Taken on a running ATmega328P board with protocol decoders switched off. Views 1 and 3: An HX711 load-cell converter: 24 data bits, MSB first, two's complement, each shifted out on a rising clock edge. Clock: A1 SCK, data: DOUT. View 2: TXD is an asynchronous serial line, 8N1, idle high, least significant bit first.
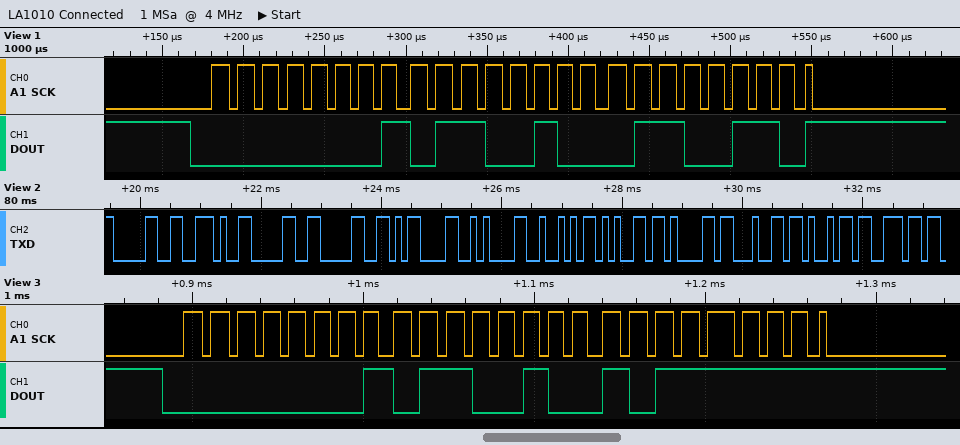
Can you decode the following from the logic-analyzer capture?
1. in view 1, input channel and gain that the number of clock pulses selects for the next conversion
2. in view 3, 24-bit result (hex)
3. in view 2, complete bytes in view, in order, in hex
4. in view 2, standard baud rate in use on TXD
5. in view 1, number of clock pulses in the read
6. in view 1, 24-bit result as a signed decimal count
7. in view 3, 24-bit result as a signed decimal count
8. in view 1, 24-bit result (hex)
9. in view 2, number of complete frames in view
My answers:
channel A, gain 128
0x0164BF
0x30 0x2E 0x30 0x30 0x0D 0x0A 0x52 0x65 0x61 0x64 0x69 0x6E
9600 baud
25
91238
91327
0x016466
12
